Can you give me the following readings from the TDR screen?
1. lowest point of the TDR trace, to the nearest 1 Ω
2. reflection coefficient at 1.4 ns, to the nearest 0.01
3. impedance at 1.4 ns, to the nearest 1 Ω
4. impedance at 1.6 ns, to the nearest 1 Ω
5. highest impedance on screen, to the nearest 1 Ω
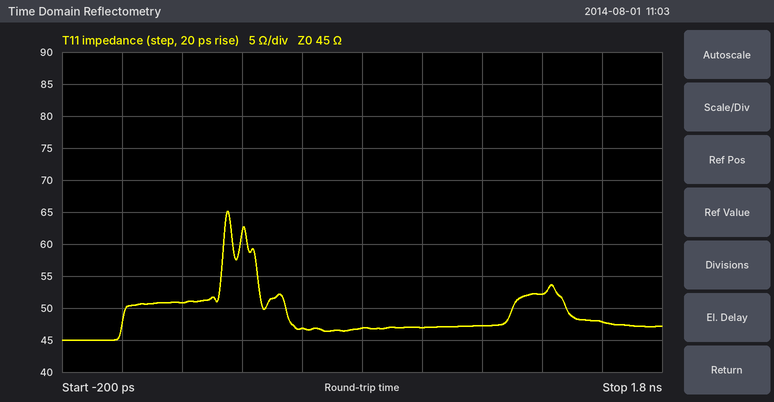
45 Ω
+0.07
52 Ω
48 Ω
65 Ω
